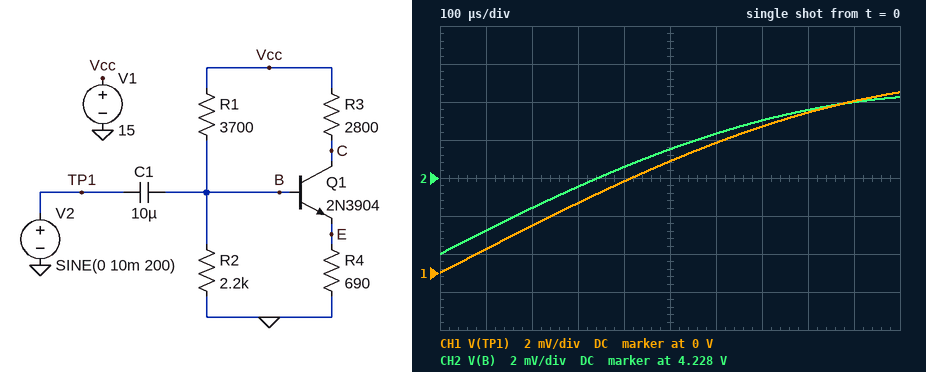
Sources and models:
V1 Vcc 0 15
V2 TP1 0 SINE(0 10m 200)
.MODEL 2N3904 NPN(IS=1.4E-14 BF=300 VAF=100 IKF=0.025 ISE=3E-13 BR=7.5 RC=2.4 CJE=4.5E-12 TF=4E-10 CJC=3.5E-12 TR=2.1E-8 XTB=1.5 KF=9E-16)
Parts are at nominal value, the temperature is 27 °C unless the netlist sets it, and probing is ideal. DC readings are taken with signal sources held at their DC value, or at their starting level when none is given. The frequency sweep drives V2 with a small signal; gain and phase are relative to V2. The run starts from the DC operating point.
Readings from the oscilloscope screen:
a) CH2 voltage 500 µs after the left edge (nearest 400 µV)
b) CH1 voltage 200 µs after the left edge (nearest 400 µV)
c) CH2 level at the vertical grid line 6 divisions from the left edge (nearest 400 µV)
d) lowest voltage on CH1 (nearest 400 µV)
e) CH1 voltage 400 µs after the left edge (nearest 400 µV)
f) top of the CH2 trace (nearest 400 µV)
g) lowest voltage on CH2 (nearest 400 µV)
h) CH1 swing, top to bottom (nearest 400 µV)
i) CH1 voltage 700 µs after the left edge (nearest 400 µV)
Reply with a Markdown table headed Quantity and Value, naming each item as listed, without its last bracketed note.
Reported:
| Quantity | Value |
|---|---|
| CH2 voltage 500 µs after the left edge | 4.2296 V |
| CH1 voltage 200 µs after the left edge | 2.4 mV |
| CH2 level at the vertical grid line 6 divisions from the left edge | 4.2304 V |
| lowest voltage on CH1 | 0 V |
| CH1 voltage 400 µs after the left edge | 4.8 mV |
| top of the CH2 trace | 4.2324 V |
| lowest voltage on CH2 | 4.2240 V |
| CH1 swing, top to bottom | 9.6 mV |
| CH1 voltage 700 µs after the left edge | 7.6 mV |
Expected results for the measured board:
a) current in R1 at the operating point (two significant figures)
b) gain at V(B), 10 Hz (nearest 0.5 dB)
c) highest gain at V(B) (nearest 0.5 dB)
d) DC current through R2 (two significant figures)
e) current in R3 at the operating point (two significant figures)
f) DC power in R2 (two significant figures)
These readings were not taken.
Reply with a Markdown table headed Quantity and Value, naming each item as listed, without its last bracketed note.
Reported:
| Quantity | Value |
|---|---|
| current in R1 at the operating point | 2.9 mA |
| gain at V(B), 10 Hz | -12.0 dB |
| highest gain at V(B) | 0 dB |
| DC current through R2 | 1.9 mA |
| current in R3 at the operating point | 4.1 mA |
| DC power in R2 | 8.1 mW |
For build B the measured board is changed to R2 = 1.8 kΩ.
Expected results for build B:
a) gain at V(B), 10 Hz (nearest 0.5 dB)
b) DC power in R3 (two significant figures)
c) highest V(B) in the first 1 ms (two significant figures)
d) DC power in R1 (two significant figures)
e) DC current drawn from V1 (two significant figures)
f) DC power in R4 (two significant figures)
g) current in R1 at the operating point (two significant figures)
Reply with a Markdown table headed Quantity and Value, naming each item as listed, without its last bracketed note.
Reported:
| Quantity | Value |
|---|---|
| gain at V(B), 10 Hz | -12.5 dB |
| DC power in R3 | 48 mW |
| highest V(B) in the first 1 ms | 4.1 V |
| DC power in R1 | 32 mW |
| DC current drawn from V1 | 7.1 mA |
| DC power in R4 | 16 mW |
| current in R1 at the operating point | 3.0 mA |
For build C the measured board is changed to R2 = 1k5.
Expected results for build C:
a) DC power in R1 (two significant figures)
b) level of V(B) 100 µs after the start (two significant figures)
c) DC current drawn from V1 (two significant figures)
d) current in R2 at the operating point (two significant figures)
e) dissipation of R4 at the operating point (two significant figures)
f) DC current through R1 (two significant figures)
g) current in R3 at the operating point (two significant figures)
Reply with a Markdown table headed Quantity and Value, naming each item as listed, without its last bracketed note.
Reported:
| Quantity | Value |
|---|---|
| DC power in R1 | 33 mW |
| level of V(B) 100 µs after the start | 3.9 V |
| DC current drawn from V1 | 7.2 mA |
| current in R2 at the operating point | 2.6 mA |
| dissipation of R4 at the operating point | 15 mW |
| DC current through R1 | 3.0 mA |
| current in R3 at the operating point | 4.2 mA |
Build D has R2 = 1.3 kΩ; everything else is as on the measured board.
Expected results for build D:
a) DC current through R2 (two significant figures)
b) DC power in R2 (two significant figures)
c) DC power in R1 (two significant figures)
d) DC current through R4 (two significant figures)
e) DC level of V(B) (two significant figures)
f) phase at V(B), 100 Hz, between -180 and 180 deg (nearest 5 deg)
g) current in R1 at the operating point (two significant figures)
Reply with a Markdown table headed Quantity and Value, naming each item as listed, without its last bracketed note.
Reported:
| Quantity | Value |
|---|---|
| DC current through R2 | 2.9 mA |
| DC power in R2 | 11 mW |
| DC power in R1 | 34 mW |
| DC current through R4 | 4.4 mA |
| DC level of V(B) | 3.7 V |
| phase at V(B), 100 Hz, between -180 and 180 deg | 25 deg |
| current in R1 at the operating point | 3.0 mA |
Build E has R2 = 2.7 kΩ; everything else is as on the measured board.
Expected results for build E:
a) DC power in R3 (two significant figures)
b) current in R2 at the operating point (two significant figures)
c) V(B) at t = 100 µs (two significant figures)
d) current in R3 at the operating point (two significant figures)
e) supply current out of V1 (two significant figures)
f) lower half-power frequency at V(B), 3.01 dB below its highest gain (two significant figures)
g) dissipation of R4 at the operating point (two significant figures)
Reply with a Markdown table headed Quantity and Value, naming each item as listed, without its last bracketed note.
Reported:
| Quantity | Value |
|---|---|
| DC power in R3 | 46 mW |
| current in R2 at the operating point | 1.6 mA |
| V(B) at t = 100 µs | 4.4 V |
| current in R3 at the operating point | 4.0 mA |
| supply current out of V1 | 6.9 mA |
| lower half-power frequency at V(B), 3.01 dB below its highest gain | 38 Hz |
| dissipation of R4 at the operating point | 19 mW |
